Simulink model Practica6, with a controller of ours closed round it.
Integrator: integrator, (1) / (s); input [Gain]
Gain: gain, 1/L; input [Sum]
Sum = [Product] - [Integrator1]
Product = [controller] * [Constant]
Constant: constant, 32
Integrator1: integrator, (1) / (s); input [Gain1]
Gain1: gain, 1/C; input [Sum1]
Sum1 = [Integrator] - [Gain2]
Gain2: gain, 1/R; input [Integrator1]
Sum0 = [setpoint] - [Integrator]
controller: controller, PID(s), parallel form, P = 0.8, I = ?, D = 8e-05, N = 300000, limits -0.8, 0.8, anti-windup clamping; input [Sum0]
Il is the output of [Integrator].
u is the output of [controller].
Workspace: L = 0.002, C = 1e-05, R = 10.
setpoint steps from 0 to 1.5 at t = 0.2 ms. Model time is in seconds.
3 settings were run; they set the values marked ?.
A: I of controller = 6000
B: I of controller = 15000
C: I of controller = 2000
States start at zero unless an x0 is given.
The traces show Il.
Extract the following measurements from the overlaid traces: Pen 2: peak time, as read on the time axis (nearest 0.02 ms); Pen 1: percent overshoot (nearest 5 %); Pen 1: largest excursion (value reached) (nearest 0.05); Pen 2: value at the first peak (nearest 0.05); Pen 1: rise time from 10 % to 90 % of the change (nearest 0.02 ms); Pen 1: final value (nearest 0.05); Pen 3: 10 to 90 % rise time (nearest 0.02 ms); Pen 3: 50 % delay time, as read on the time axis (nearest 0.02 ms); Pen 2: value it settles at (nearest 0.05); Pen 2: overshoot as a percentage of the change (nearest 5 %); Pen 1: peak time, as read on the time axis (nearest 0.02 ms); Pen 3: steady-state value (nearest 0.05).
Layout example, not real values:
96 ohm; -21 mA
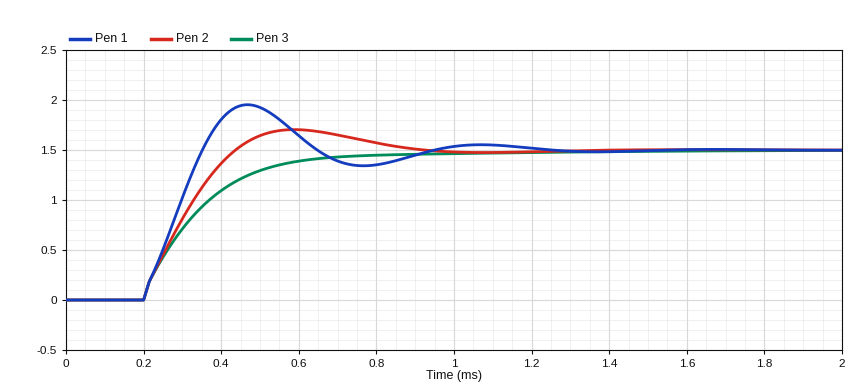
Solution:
0.58 ms; 30 %; 1.95; 1.70; 0.12 ms; 1.50; 0.34 ms; 0.30 ms; 1.50; 15 %; 0.46 ms; 1.50
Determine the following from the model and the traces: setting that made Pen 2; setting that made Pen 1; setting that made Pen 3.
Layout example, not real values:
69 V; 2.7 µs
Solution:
A; B; C
